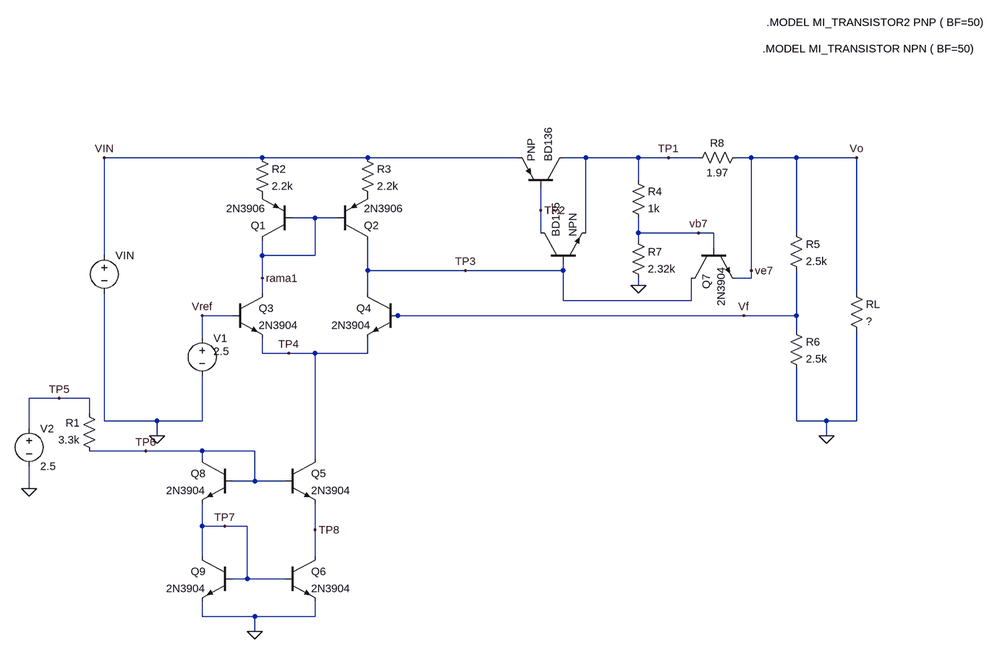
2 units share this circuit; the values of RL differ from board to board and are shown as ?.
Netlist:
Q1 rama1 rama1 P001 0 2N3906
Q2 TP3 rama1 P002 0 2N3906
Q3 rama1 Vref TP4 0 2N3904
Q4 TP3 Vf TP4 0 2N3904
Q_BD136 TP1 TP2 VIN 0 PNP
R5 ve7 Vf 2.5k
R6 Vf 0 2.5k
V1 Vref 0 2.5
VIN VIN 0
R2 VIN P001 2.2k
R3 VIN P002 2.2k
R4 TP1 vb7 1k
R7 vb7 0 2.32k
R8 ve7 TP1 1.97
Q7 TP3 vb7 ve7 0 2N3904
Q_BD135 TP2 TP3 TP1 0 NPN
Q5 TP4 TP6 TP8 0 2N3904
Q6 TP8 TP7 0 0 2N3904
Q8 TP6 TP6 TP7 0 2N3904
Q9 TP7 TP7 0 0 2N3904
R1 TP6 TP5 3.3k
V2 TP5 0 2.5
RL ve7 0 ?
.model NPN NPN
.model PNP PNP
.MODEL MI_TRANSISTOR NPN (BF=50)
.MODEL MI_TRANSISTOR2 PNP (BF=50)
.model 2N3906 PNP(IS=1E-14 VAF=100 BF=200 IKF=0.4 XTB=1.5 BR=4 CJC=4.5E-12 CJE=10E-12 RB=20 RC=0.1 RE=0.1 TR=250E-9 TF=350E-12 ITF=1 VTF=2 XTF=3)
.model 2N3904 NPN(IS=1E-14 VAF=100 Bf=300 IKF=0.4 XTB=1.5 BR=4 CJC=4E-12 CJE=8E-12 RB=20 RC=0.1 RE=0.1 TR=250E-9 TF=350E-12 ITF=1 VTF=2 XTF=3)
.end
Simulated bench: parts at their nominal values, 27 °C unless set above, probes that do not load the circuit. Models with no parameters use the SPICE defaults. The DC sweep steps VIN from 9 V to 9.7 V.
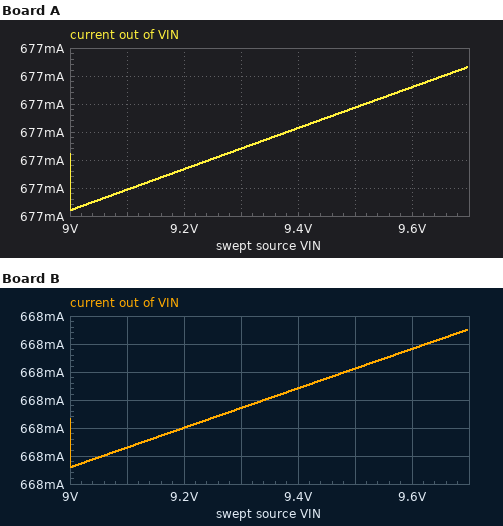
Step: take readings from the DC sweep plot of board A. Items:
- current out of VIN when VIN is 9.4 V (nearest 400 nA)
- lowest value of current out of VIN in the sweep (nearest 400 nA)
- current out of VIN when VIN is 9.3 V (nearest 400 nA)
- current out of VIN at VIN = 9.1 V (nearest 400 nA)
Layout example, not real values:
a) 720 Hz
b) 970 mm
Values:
a) 676.5164 mA
b) 676.5104 mA
c) 676.5148 mA
d) 676.5120 mA
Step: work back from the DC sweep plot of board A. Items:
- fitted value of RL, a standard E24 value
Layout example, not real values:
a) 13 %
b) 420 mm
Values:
a) 1.5 Ω
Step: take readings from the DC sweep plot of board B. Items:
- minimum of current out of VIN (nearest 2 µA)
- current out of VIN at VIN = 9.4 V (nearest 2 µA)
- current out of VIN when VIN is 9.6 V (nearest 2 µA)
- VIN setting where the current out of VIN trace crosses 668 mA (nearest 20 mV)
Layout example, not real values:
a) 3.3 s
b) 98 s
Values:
a) 667.566 mA
b) 667.594 mA
c) 667.608 mA
d) 9.34 V
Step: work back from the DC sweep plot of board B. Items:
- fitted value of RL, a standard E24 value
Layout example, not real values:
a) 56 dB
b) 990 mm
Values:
a) 7.5 Ω
